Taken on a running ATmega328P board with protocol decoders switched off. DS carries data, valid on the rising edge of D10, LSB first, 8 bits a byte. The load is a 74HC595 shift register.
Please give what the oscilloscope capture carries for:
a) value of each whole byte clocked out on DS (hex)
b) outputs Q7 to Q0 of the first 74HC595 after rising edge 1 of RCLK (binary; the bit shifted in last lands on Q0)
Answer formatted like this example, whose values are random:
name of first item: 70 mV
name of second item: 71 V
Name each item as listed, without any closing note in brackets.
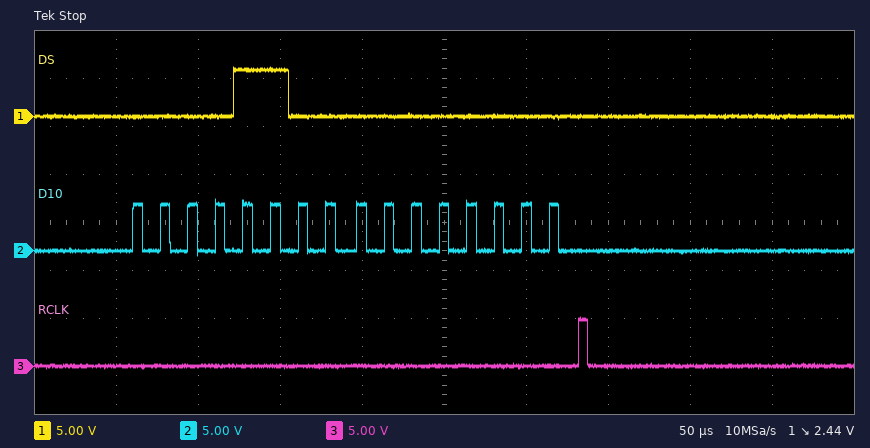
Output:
value of each whole byte clocked out on DS: 30 00
outputs Q7 to Q0 of the first 74HC595 after rising edge 1 of RCLK: 00000000
